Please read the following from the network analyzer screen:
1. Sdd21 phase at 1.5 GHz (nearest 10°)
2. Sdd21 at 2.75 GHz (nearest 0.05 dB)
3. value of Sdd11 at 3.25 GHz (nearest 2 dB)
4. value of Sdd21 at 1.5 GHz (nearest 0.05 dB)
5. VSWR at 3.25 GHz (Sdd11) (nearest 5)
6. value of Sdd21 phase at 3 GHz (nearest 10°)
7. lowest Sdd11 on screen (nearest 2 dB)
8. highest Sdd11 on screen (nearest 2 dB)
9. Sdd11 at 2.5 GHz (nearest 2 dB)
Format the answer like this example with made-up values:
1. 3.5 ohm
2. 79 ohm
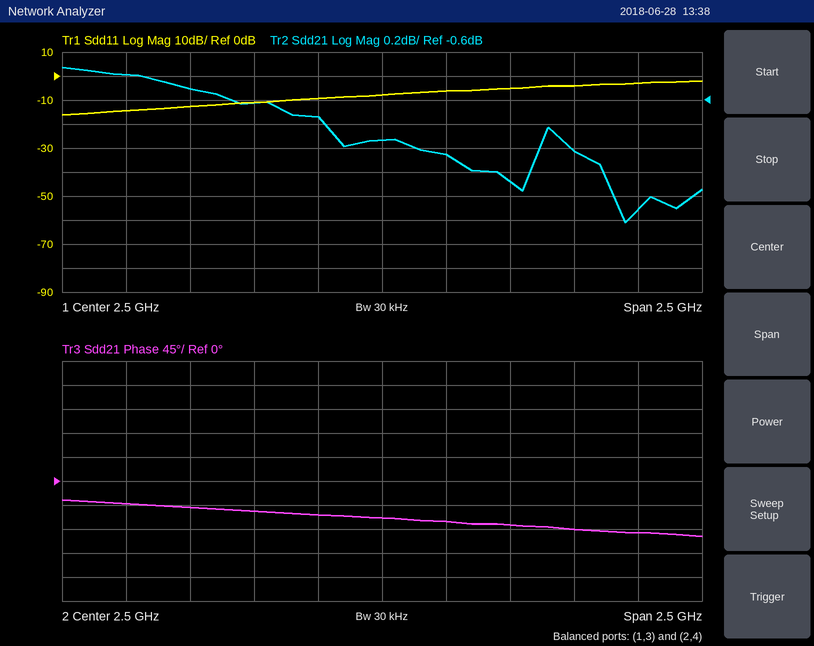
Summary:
1. -40°
2. -1.05 dB
3. -4 dB
4. -0.40 dB
5. 5
6. -80°
7. -16 dB
8. -2 dB
9. -8 dB
